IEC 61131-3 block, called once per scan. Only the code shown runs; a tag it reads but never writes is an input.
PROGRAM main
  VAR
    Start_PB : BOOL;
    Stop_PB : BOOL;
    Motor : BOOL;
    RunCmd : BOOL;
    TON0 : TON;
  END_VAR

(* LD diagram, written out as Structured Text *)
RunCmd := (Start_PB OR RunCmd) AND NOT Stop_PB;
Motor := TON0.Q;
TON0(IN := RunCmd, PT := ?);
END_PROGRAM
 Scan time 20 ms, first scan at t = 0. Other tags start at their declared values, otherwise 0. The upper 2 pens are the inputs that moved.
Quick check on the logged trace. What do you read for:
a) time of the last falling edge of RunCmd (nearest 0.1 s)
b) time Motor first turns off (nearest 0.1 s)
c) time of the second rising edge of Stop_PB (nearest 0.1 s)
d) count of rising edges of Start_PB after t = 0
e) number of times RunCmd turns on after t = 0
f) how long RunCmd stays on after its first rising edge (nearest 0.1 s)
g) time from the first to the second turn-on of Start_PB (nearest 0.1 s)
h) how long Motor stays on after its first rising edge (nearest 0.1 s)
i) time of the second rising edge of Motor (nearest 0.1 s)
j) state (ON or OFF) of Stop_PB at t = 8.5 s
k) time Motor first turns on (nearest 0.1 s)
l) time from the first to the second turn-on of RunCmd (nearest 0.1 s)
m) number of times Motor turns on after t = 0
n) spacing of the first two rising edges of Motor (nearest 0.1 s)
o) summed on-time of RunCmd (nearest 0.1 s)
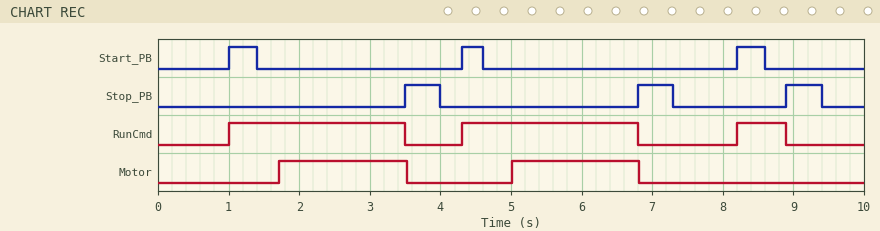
8.9 s
3.5 s
6.8 s
3
3
2.5 s
3.3 s
1.8 s
5.0 s
OFF
1.7 s
3.3 s
2
3.3 s
5.7 s
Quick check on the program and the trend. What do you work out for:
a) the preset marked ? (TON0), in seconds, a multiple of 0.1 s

0.7 s
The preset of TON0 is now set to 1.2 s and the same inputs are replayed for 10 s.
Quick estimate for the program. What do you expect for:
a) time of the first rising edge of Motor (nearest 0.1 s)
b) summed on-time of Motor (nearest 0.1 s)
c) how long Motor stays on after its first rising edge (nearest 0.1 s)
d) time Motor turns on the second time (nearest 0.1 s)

2.2 s
2.6 s
1.3 s
5.5 s
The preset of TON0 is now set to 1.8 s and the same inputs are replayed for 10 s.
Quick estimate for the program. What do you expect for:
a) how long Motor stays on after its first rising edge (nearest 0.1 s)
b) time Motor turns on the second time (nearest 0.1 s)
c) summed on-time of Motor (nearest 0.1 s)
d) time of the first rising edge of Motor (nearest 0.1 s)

0.7 s
6.1 s
1.4 s
2.8 s
